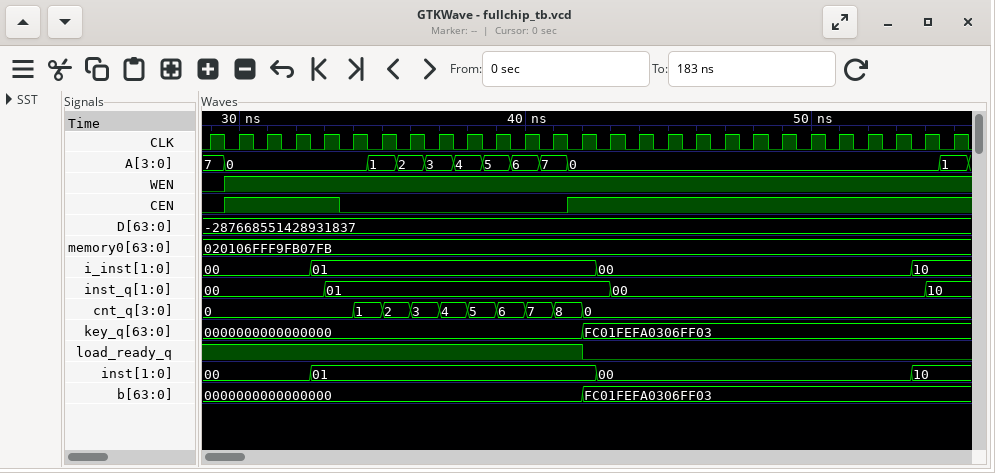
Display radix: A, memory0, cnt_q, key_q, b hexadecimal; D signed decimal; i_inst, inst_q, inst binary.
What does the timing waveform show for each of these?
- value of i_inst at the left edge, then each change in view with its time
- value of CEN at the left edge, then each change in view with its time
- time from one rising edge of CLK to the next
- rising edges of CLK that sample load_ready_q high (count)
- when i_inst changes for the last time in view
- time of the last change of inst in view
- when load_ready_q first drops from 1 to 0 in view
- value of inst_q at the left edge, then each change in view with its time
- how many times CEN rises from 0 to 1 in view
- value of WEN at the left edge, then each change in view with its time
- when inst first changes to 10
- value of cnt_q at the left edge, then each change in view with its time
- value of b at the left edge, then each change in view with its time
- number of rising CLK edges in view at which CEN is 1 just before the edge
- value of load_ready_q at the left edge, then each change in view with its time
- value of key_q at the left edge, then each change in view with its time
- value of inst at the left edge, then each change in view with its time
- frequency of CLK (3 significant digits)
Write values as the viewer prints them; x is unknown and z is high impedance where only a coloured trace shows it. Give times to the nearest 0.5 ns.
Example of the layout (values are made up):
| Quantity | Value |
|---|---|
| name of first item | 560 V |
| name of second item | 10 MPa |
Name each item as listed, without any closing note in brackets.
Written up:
| Quantity | Value |
|---|---|
| value of i_inst at the left edge, then each change in view with its time | 00, 01 at 32.5 ns, 00 at 42.5 ns, 10 at 53.5 ns |
| value of CEN at the left edge, then each change in view with its time | 0, 1 at 29.5 ns, 0 at 33.5 ns, 1 at 41.5 ns |
| time from one rising edge of CLK to the next | 1 ns |
| rising edges of CLK that sample load_ready_q high | 14 |
| when i_inst changes for the last time in view | 53.5 ns |
| time of the last change of inst in view | 53.5 ns |
| when load_ready_q first drops from 1 to 0 in view | 42 ns |
| value of inst_q at the left edge, then each change in view with its time | 00, 01 at 33 ns, 00 at 43 ns, 10 at 54 ns |
| how many times CEN rises from 0 to 1 in view | 2 |
| value of WEN at the left edge, then each change in view with its time | 0, 1 at 29.5 ns |
| when inst first changes to 10 | 53.5 ns |
| value of cnt_q at the left edge, then each change in view with its time | 0, 1 at 34 ns, 2 at 35 ns, 3 at 36 ns, 4 at 37 ns, 5 at 38 ns, 6 at 39 ns, 7 at 40 ns, 8 at 41 ns, 0 at 42 ns |
| value of b at the left edge, then each change in view with its time | 0000000000000000, FC01FEFA0306FF03 at 42 ns |
| number of rising CLK edges in view at which CEN is 1 just before the edge | 18 |
| value of load_ready_q at the left edge, then each change in view with its time | 1, 0 at 42 ns |
| value of key_q at the left edge, then each change in view with its time | 0000000000000000, FC01FEFA0306FF03 at 42 ns |
| value of inst at the left edge, then each change in view with its time | 00, 01 at 32.5 ns, 00 at 42.5 ns, 10 at 53.5 ns |
| frequency of CLK | 1.00 GHz |
